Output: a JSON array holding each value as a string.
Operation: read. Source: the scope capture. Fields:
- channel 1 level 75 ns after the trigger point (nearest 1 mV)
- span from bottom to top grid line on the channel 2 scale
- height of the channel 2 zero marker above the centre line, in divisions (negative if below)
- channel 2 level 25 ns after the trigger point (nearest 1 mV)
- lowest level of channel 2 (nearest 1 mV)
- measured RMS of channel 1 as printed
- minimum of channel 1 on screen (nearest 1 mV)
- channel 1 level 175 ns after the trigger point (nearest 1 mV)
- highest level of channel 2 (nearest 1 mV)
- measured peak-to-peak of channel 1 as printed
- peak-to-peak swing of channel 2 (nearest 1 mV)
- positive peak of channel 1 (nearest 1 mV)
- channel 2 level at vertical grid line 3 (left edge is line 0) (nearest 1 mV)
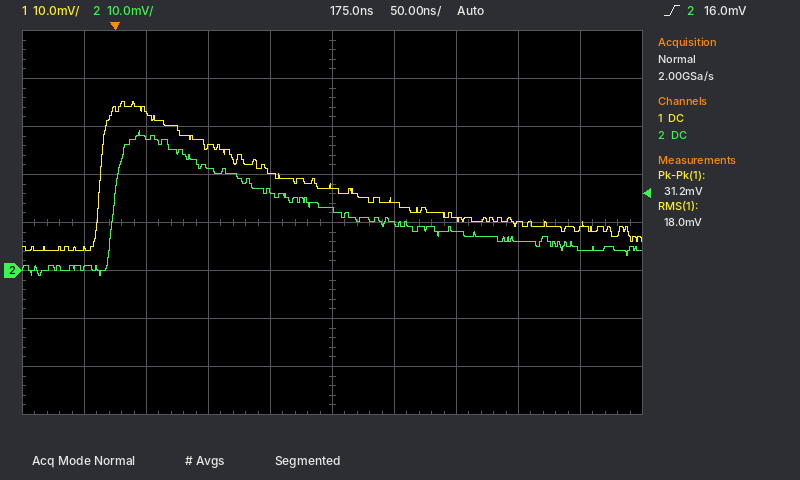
["26 mV", "80 mV", "-1.0 div", "28 mV", "-1 mV", "18.0 mV", "4 mV", "18 mV", "29 mV", "31.2 mV", "30 mV", "35 mV", "22 mV"]
